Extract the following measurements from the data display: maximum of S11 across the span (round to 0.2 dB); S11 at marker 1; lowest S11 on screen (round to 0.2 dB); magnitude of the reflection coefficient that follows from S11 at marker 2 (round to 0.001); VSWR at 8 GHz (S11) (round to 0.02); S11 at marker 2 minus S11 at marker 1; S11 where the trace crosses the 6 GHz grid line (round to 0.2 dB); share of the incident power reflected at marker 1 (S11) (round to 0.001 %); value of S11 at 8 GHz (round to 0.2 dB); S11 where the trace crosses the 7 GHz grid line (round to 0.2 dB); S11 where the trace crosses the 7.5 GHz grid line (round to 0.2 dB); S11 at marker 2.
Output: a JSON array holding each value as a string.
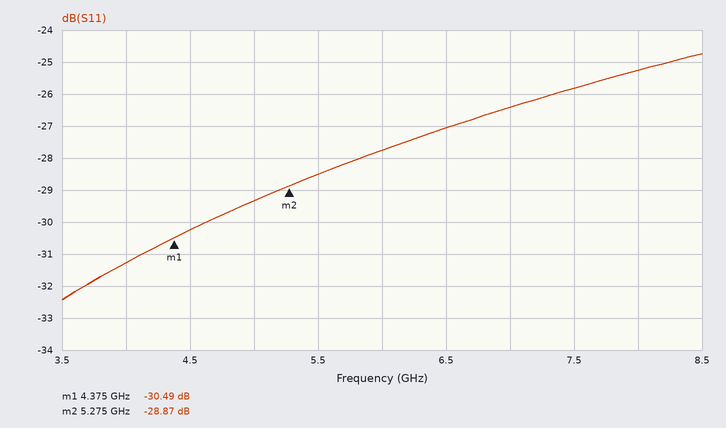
["-24.8 dB", "-30.49 dB", "-32.4 dB", "0.036", "1.12", "1.62 dB", "-27.8 dB", "0.089 %", "-25.2 dB", "-26.4 dB", "-25.8 dB", "-28.87 dB"]
